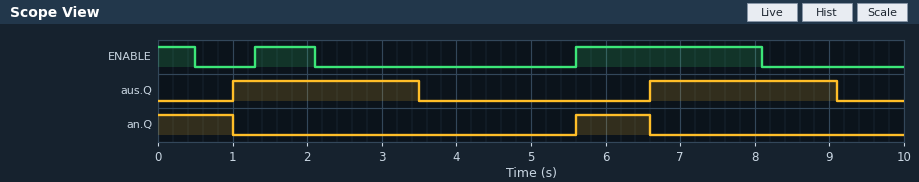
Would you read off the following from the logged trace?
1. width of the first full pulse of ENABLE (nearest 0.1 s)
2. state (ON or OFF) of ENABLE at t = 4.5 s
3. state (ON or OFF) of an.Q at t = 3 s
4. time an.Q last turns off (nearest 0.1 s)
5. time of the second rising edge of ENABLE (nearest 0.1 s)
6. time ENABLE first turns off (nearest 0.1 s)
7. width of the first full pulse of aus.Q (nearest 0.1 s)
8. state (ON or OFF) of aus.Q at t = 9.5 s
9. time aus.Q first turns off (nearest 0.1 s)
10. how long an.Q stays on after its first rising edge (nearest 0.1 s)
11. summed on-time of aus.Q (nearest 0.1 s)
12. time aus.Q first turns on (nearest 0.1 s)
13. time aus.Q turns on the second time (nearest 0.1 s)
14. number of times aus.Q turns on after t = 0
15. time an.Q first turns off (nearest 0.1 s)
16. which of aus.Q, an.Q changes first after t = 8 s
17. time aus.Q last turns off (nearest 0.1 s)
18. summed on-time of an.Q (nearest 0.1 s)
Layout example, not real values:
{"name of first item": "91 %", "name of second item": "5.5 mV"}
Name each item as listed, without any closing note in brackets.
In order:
{"width of the first full pulse of ENABLE": "0.8 s", "state (ON or OFF) of ENABLE at t = 4.5 s": "OFF", "state (ON or OFF) of an.Q at t = 3 s": "OFF", "time an.Q last turns off": "6.6 s", "time of the second rising edge of ENABLE": "5.6 s", "time ENABLE first turns off": "0.5 s", "width of the first full pulse of aus.Q": "2.5 s", "state (ON or OFF) of aus.Q at t = 9.5 s": "OFF", "time aus.Q first turns off": "3.5 s", "how long an.Q stays on after its first rising edge": "1.0 s", "summed on-time of aus.Q": "5.0 s", "time aus.Q first turns on": "1.0 s", "time aus.Q turns on the second time": "6.6 s", "number of times aus.Q turns on after t = 0": "2", "time an.Q first turns off": "1.0 s", "which of aus.Q, an.Q changes first after t = 8 s": "aus.Q", "time aus.Q last turns off": "9.1 s", "summed on-time of an.Q": "2.0 s"}
